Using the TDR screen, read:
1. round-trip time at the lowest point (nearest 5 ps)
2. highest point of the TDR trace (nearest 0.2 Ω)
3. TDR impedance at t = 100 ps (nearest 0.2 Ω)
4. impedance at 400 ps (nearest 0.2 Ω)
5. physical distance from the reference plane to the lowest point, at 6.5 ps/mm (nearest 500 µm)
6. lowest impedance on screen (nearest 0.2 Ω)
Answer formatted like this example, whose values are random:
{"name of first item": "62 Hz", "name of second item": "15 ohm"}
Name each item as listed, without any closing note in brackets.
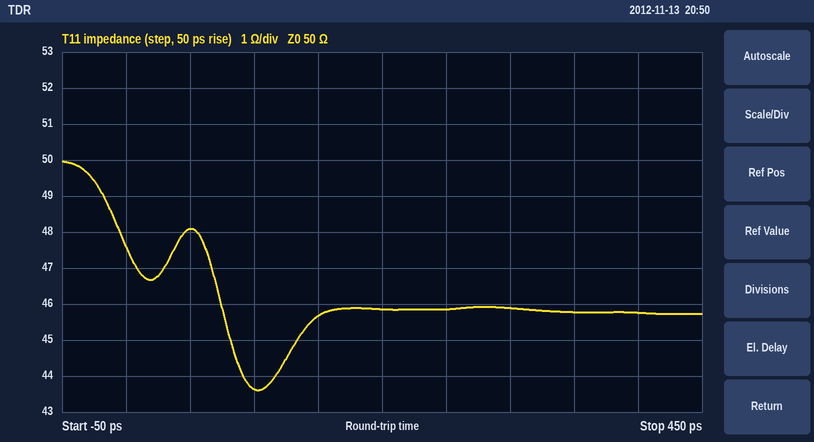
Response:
{"round-trip time at the lowest point": "105 ps", "highest point of the TDR trace": "50.0 Ω", "TDR impedance at t = 100 ps": "43.6 Ω", "impedance at 400 ps": "45.8 Ω", "physical distance from the reference plane to the lowest point, at 6.5 ps/mm": "8.0 mm", "lowest impedance on screen": "43.6 Ω"}
